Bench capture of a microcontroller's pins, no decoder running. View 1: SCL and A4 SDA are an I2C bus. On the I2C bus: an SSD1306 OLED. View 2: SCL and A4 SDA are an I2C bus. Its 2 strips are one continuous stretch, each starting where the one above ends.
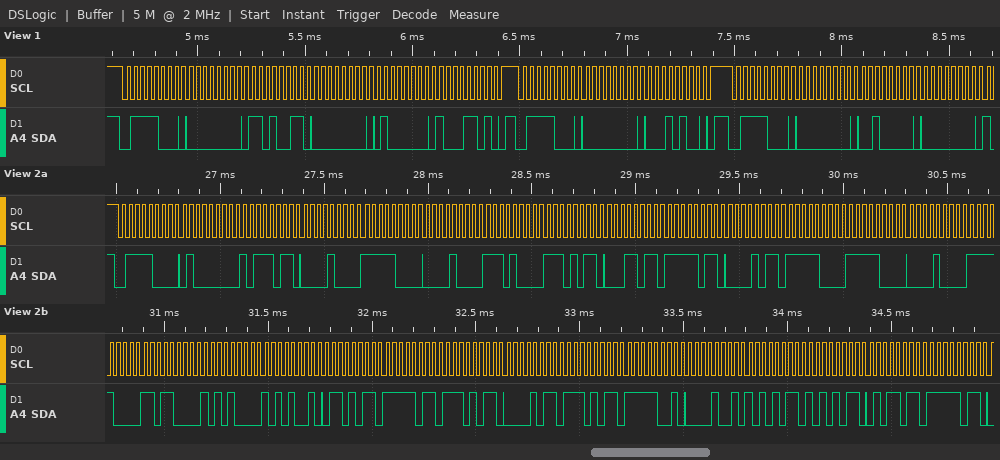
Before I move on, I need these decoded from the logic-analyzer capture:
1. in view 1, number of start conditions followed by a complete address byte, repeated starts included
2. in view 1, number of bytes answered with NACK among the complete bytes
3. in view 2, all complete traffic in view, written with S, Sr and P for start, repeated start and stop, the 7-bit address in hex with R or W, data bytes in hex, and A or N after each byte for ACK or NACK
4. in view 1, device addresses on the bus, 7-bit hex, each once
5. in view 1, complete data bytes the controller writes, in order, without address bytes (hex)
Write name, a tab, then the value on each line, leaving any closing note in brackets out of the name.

in view 1, number of start conditions followed by a complete address byte, repeated starts included	3
in view 1, number of bytes answered with NACK among the complete bytes	0
in view 2, all complete traffic in view, written with S, Sr and P for start, repeated start and stop, the 7-bit address in hex with R or W, data bytes in hex, and A or N after each byte for ACK or NACK	S 3CW A 40 A BB A 08 A F8 A 08 A E8 A EB A 1B A FB A 0B A F8 A F8 A 08 A F8 A D8 A A8 A A9 A 6B A FB A EB A 0B A EB A F9 A 09 A AB A AB A 5B A FB A
in view 1, device addresses on the bus, 7-bit hex, each once	0x3C
in view 1, complete data bytes the controller writes, in order, without address bytes	00 D3 00 40 8D 00 14 00 20 00
